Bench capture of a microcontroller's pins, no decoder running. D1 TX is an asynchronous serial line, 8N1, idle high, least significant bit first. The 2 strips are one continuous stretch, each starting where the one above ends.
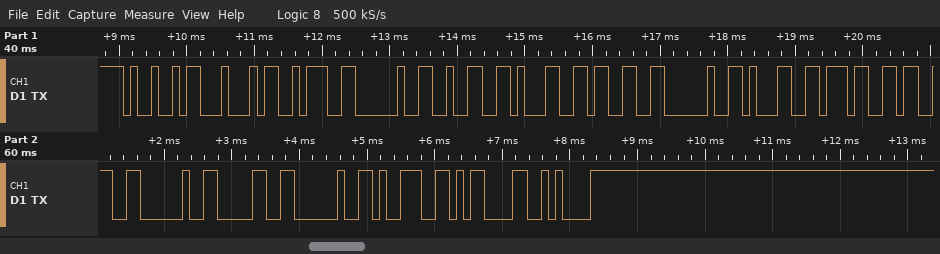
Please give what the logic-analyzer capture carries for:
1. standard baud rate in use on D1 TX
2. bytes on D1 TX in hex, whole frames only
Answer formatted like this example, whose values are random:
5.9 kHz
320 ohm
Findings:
9600 baud
49 44 3A 20 32 31 33 20 31 37 33 20 30 20 39 0D 0A
